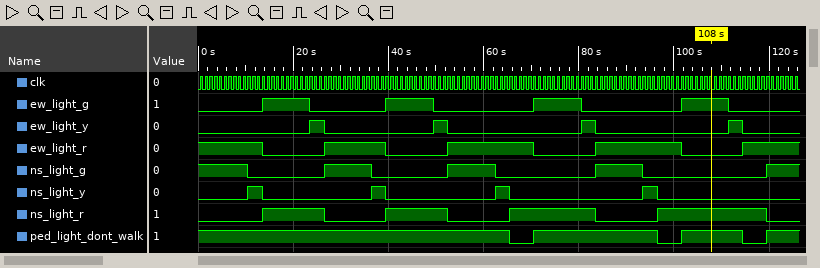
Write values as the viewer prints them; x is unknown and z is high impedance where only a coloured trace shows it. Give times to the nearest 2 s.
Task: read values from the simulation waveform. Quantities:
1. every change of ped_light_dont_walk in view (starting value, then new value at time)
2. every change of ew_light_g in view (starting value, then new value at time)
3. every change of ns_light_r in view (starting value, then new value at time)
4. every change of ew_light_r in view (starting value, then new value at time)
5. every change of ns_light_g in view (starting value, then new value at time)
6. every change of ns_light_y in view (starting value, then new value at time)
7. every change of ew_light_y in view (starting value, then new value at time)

1, 0 at 66 s, 1 at 70 s, 0 at 96 s, 1 at 102 s, 0 at 114 s, 1 at 120 s
0, 1 at 14 s, 0 at 24 s, 1 at 40 s, 0 at 50 s, 1 at 70 s, 0 at 80 s, 1 at 102 s, 0 at 112 s
0, 1 at 14 s, 0 at 26 s, 1 at 40 s, 0 at 52 s, 1 at 66 s, 0 at 84 s, 1 at 96 s, 0 at 120 s
1, 0 at 14 s, 1 at 26 s, 0 at 40 s, 1 at 52 s, 0 at 70 s, 1 at 84 s, 0 at 102 s, 1 at 114 s
1, 0 at 10 s, 1 at 26 s, 0 at 36 s, 1 at 52 s, 0 at 62 s, 1 at 84 s, 0 at 94 s, 1 at 120 s
0, 1 at 10 s, 0 at 14 s, 1 at 36 s, 0 at 40 s, 1 at 62 s, 0 at 66 s, 1 at 94 s, 0 at 96 s
0, 1 at 24 s, 0 at 26 s, 1 at 50 s, 0 at 52 s, 1 at 80 s, 0 at 84 s, 1 at 112 s, 0 at 114 s
